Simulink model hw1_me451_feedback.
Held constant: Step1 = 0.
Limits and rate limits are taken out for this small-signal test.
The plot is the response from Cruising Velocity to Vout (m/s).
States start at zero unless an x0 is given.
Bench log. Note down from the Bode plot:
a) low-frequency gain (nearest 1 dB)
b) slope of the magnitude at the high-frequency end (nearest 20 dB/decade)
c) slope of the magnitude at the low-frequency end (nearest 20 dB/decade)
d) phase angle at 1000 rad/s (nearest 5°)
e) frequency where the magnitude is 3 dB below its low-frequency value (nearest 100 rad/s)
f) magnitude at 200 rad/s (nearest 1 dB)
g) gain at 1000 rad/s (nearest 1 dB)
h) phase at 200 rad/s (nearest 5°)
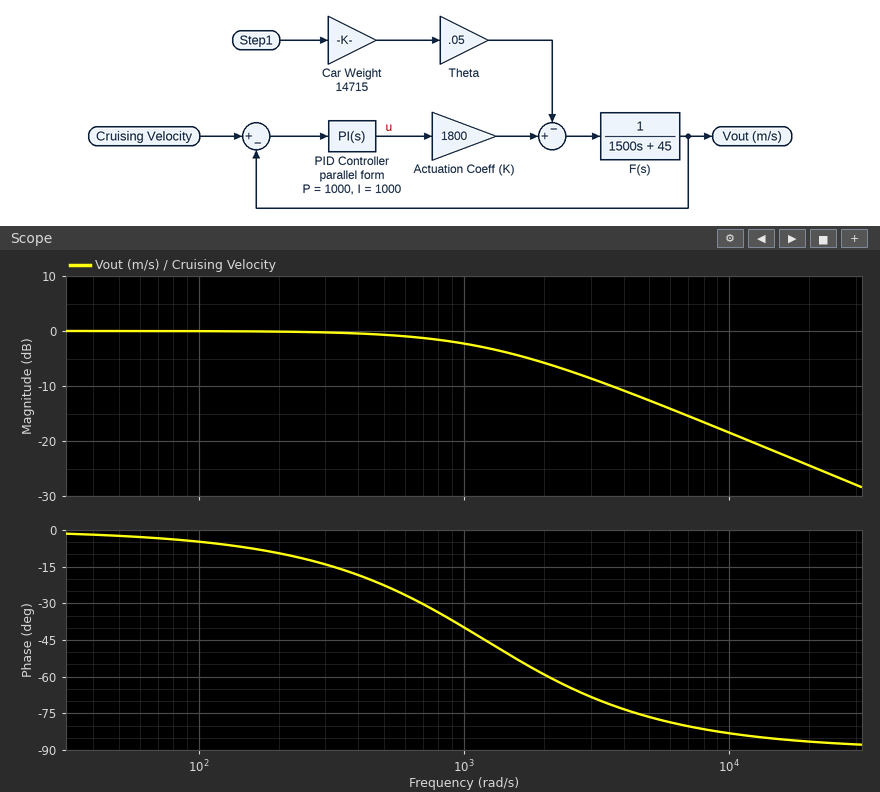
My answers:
0 dB
-20 dB/decade
0 dB/decade
-40°
1200 rad/s
0 dB
-2 dB
-10°
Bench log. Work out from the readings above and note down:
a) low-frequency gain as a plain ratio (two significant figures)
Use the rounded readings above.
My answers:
1.0
